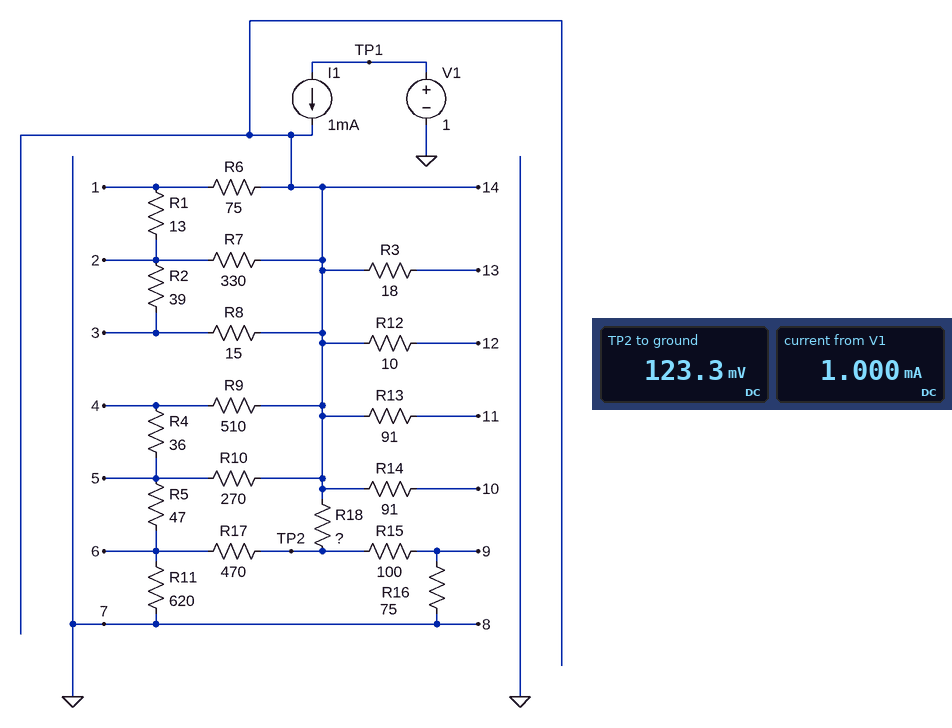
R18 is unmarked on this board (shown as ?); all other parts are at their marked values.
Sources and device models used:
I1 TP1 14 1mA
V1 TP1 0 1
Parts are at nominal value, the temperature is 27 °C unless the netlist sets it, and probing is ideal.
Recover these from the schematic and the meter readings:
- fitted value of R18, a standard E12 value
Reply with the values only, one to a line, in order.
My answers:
270 Ω
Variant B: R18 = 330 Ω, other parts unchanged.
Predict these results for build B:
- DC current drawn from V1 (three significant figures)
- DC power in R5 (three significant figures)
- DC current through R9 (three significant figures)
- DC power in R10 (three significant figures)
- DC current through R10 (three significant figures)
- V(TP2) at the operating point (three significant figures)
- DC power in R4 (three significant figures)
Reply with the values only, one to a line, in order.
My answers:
1.00 mA
10.1 µW
153 µA
25.9 µW
310 µA
121 mV
845 nW
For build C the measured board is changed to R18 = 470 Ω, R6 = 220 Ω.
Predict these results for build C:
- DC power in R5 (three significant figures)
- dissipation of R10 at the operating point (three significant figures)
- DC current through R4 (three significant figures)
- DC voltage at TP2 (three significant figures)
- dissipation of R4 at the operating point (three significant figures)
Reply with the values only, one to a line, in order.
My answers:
13.6 µW
35.1 µW
178 µA
116 mV
1.14 µW
